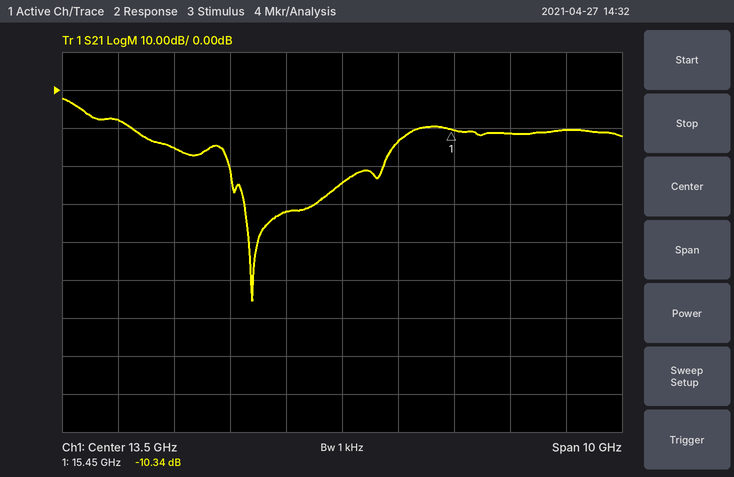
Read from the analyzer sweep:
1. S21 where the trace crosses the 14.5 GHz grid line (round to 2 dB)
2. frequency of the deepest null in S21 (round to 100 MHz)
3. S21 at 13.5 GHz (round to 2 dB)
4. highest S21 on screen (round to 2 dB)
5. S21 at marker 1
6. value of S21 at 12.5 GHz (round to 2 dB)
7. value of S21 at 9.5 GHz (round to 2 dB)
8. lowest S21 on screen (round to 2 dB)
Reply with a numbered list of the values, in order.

1. -14 dB
2. 11.9 GHz
3. -24 dB
4. -2 dB
5. -10.34 dB
6. -32 dB
7. -8 dB
8. -56 dB
